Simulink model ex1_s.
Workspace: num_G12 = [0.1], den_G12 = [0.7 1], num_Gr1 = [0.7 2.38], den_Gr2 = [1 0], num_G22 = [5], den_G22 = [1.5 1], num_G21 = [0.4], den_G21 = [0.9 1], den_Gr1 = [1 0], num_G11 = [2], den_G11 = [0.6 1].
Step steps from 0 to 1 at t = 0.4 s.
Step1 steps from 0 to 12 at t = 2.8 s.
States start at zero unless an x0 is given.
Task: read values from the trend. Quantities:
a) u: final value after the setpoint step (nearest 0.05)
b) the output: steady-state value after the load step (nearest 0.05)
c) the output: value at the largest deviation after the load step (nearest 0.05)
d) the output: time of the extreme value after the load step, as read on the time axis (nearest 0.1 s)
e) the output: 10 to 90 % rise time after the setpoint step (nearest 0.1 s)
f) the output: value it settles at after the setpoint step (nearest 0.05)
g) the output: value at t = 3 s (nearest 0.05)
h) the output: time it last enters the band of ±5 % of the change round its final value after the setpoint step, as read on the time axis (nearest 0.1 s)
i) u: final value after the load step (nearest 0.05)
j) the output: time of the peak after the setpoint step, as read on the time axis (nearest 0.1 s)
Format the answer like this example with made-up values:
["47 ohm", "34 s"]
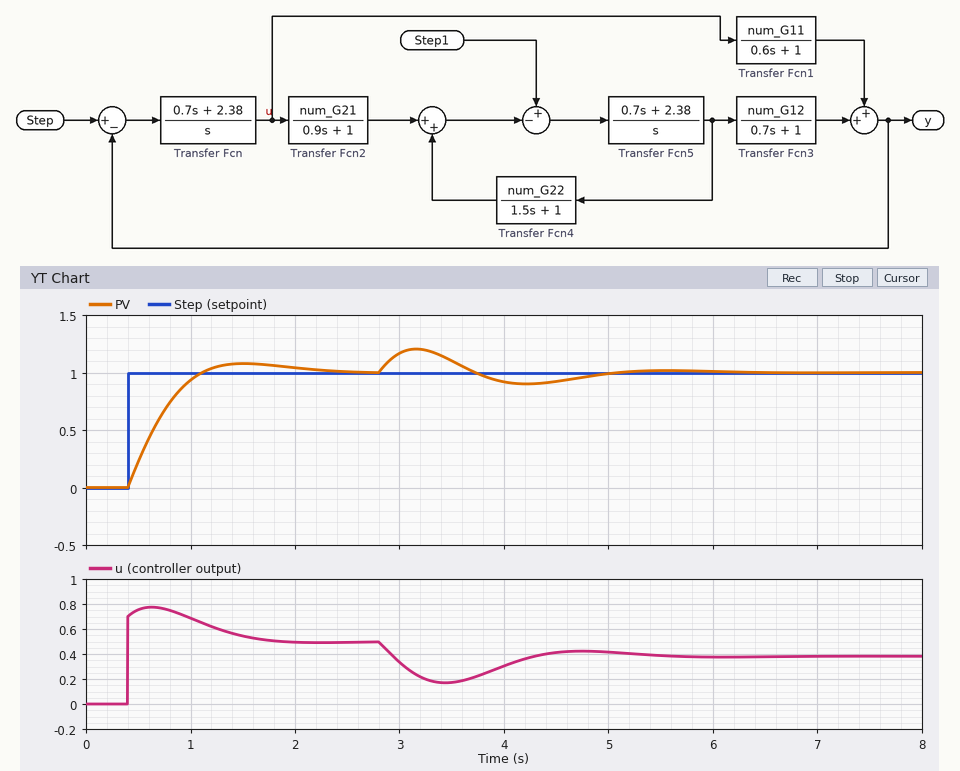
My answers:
["0.50", "1.00", "1.20", "3.2 s", "0.5 s", "1.00", "1.15", "1.9 s", "0.40", "1.5 s"]
